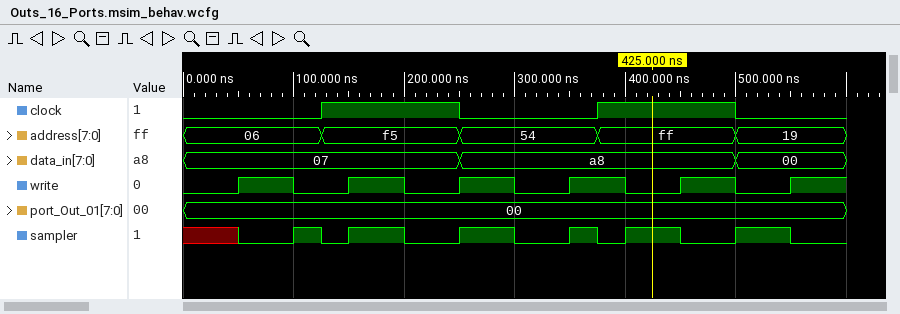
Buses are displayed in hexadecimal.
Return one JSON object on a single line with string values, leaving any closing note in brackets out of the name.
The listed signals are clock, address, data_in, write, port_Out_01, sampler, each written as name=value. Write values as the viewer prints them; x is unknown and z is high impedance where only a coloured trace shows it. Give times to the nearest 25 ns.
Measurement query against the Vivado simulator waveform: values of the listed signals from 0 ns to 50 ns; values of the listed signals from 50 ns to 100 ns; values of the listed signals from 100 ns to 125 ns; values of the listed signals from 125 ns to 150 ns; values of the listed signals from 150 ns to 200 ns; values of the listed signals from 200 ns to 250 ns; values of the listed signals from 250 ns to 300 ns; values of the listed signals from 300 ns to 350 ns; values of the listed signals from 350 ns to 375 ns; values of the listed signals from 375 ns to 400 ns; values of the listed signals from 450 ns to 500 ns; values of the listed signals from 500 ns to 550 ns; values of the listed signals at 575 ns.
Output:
{"values of the listed signals from 0 ns to 50 ns": "clock=0, address=06, data_in=07, write=0, port_Out_01=00, sampler=x", "values of the listed signals from 50 ns to 100 ns": "clock=0, address=06, data_in=07, write=1, port_Out_01=00, sampler=0", "values of the listed signals from 100 ns to 125 ns": "clock=0, address=06, data_in=07, write=0, port_Out_01=00, sampler=1", "values of the listed signals from 125 ns to 150 ns": "clock=1, address=f5, data_in=07, write=0, port_Out_01=00, sampler=0", "values of the listed signals from 150 ns to 200 ns": "clock=1, address=f5, data_in=07, write=1, port_Out_01=00, sampler=1", "values of the listed signals from 200 ns to 250 ns": "clock=1, address=f5, data_in=07, write=0, port_Out_01=00, sampler=0", "values of the listed signals from 250 ns to 300 ns": "clock=0, address=54, data_in=a8, write=1, port_Out_01=00, sampler=1", "values of the listed signals from 300 ns to 350 ns": "clock=0, address=54, data_in=a8, write=0, port_Out_01=00, sampler=0", "values of the listed signals from 350 ns to 375 ns": "clock=0, address=54, data_in=a8, write=1, port_Out_01=00, sampler=1", "values of the listed signals from 375 ns to 400 ns": "clock=1, address=ff, data_in=a8, write=1, port_Out_01=00, sampler=0", "values of the listed signals from 450 ns to 500 ns": "clock=1, address=ff, data_in=a8, write=1, port_Out_01=00, sampler=0", "values of the listed signals from 500 ns to 550 ns": "clock=0, address=19, data_in=00, write=0, port_Out_01=00, sampler=1", "values of the listed signals at 575 ns": "clock=0, address=19, data_in=00, write=1, port_Out_01=00, sampler=0"}
